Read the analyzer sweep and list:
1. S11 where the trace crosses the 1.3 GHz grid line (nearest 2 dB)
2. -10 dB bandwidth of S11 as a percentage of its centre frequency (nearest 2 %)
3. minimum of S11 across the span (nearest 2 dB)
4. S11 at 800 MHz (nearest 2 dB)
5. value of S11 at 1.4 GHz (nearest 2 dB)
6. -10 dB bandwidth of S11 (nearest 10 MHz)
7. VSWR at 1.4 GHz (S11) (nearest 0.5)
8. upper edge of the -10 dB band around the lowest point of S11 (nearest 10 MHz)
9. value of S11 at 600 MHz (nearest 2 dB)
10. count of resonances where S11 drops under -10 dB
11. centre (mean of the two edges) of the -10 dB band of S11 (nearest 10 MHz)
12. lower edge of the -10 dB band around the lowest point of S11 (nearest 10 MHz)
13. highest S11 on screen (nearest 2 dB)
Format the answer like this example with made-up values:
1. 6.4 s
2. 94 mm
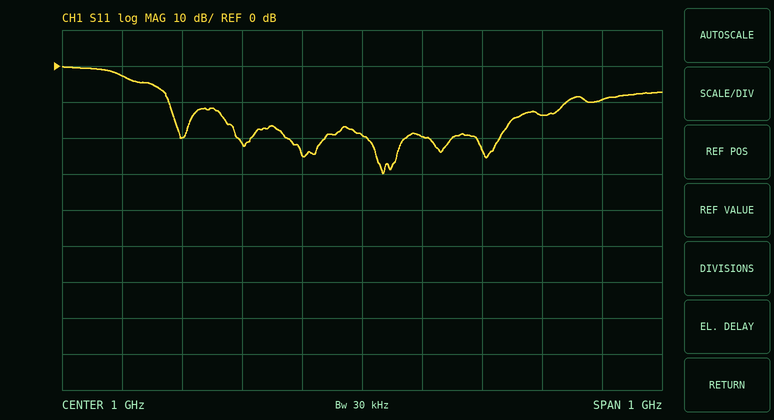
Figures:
1. -14 dB
2. 66 %
3. -30 dB
4. -22 dB
5. -10 dB
6. 660 MHz
7. 2.0
8. 1.34 GHz
9. -2 dB
10. 6
11. 1.01 GHz
12. 680 MHz
13. 0 dB
